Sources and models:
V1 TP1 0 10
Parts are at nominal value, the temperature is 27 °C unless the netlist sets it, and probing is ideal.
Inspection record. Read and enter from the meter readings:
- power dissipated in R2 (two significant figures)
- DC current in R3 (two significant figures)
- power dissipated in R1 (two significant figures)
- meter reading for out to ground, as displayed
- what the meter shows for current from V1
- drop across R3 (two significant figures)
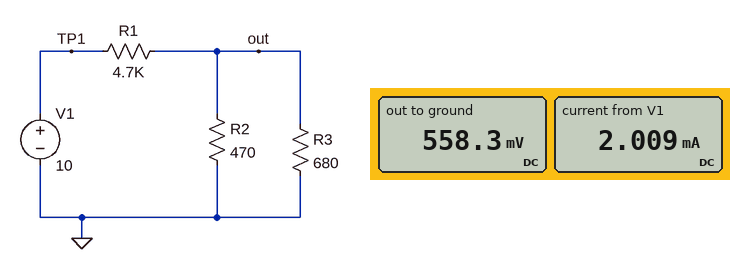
660 µW
820 µA
19 mW
558.3 mV
2.009 mA
560 mV
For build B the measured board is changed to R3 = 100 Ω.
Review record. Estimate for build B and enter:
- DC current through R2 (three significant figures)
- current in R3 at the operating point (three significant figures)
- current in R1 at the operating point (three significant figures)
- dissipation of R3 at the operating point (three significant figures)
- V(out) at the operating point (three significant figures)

367 µA
1.72 mA
2.09 mA
297 µW
172 mV
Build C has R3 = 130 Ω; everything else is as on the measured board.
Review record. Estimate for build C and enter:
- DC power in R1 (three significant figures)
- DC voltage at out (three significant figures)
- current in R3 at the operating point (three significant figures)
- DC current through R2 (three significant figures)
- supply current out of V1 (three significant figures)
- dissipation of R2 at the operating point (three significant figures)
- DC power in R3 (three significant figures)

20.4 mW
212 mV
1.63 mA
451 µA
2.08 mA
95.7 µW
346 µW
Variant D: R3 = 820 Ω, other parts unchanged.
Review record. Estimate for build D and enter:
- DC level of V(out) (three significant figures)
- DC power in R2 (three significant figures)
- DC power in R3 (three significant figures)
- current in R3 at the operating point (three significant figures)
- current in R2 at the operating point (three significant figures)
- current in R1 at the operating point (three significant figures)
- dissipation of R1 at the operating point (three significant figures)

598 mV
760 µW
436 µW
729 µA
1.27 mA
2.00 mA
18.8 mW
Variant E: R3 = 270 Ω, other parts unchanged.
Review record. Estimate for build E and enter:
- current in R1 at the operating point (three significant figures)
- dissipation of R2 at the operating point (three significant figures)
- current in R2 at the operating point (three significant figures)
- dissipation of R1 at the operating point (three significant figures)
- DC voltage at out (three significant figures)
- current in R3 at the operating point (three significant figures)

2.05 mA
264 µW
749 µA
19.8 mW
352 mV
1.30 mA
